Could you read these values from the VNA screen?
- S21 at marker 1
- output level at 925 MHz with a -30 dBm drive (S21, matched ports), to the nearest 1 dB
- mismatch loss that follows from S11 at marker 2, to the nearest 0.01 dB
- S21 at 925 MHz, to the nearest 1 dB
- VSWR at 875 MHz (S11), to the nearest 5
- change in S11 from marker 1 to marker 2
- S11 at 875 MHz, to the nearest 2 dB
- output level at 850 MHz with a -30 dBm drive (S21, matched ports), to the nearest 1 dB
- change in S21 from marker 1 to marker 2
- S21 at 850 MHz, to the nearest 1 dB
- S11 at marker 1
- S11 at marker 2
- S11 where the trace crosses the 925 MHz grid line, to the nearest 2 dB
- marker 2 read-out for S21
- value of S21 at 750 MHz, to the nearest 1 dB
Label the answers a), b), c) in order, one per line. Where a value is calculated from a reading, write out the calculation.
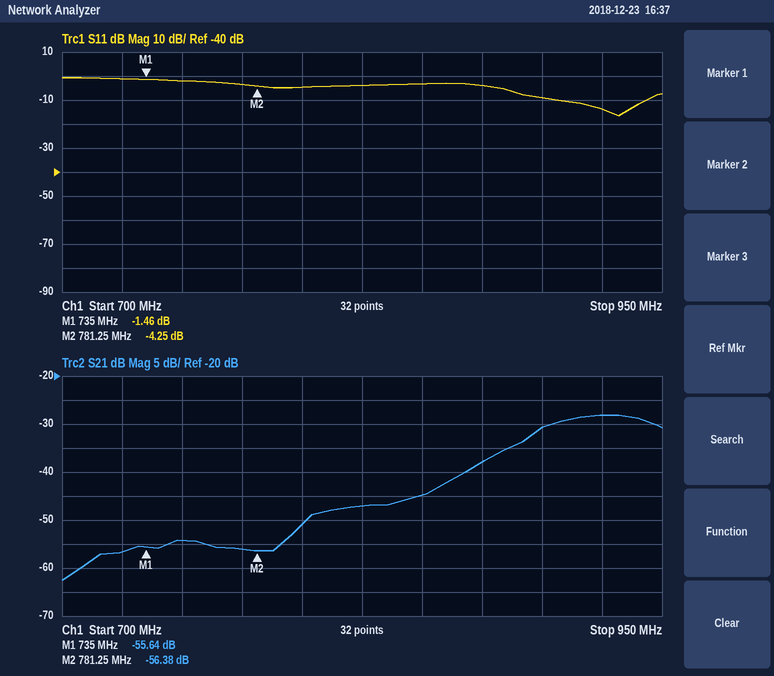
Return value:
a) -55.64 dB
b) -30 dBm + (-28 dB) = -58 dBm
c) −10 log10(1 − 10^(-4.25/10)) ≈ 2.05 dB
d) -28 dB
e) |Γ| = 10^(-4/20) = 0.6310; VSWR = (1 + 0.6310)/(1 − 0.6310) ≈ 4.42, so 5 to the nearest 5
f) -4.25 − (-1.46) = -2.79 dB
g) -4 dB
h) -30 dBm + (-45 dB) = -75 dBm
i) -56.38 − (-55.64) = -0.74 dB
j) -45 dB
k) -1.46 dB
l) -4.25 dB
m) -14 dB
n) -56.38 dB
o) -54 dB
